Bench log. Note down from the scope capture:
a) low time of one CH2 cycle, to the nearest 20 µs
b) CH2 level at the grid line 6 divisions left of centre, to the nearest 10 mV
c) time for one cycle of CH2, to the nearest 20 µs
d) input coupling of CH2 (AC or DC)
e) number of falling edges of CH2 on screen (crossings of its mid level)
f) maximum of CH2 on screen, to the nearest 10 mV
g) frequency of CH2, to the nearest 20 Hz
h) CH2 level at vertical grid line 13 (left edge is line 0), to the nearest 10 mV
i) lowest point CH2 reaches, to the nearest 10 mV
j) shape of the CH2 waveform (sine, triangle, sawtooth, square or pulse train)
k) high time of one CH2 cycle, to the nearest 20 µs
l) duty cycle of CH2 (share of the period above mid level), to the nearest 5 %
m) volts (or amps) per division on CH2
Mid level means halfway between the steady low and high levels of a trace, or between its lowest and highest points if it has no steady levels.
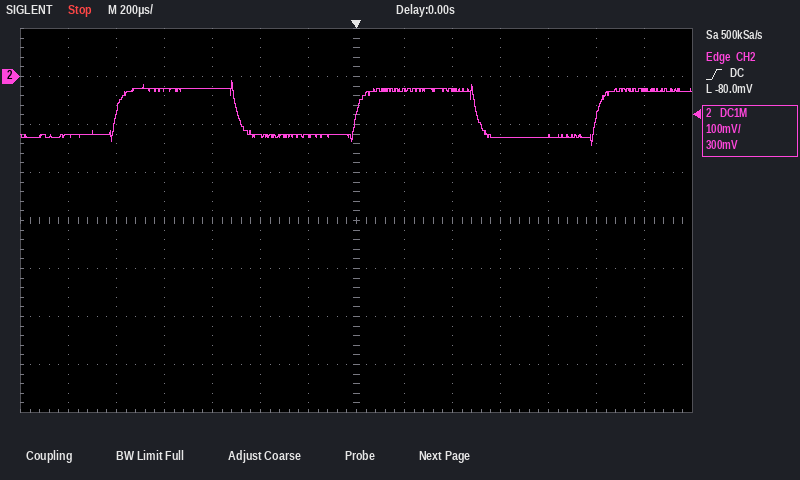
500 µs
-120 mV
1.00 ms
DC
2
-10 mV
1.00 kHz
-30 mV
-140 mV
square
500 µs
50 %
100 mV
